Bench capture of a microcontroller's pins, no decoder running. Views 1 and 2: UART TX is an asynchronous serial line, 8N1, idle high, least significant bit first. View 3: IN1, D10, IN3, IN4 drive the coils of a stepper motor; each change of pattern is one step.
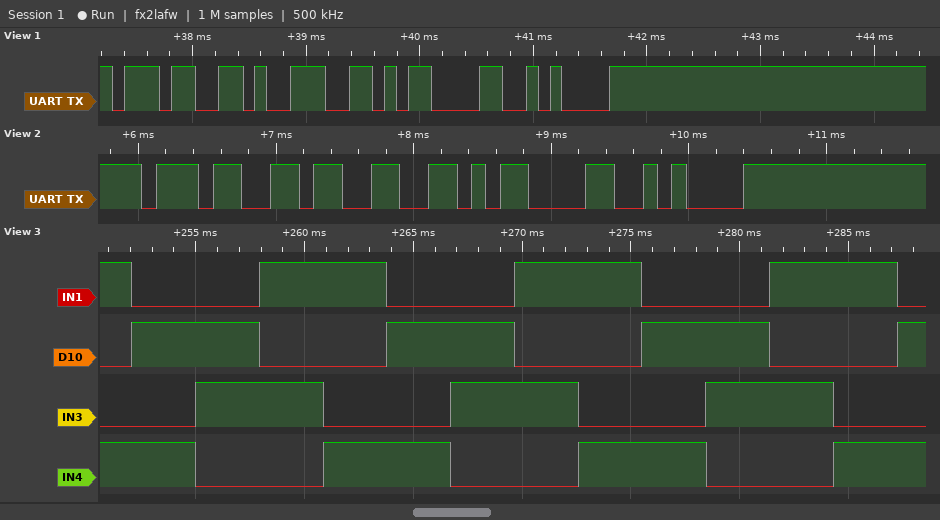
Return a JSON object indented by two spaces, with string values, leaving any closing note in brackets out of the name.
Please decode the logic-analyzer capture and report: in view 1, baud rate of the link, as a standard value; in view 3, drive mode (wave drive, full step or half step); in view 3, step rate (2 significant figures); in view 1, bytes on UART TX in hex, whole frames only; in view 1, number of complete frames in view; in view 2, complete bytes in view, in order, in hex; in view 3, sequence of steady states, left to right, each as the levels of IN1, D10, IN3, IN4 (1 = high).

{
  "in view 1, baud rate of the link, as a standard value": "9600 baud",
  "in view 3, drive mode": "full step",
  "in view 3, step rate": "340 steps/s",
  "in view 1, bytes on UART TX in hex, whole frames only": "37 39 0D 0A",
  "in view 1, number of complete frames in view": "4",
  "in view 2, complete bytes in view, in order, in hex": "37 33 0D 0A",
  "in view 3, sequence of steady states, left to right, each as the levels of IN1, D10, IN3, IN4": "1001 0101 0110 1010 1001 0101 0110 1010 1001 0101 0110 1010 1001 0101"
}
